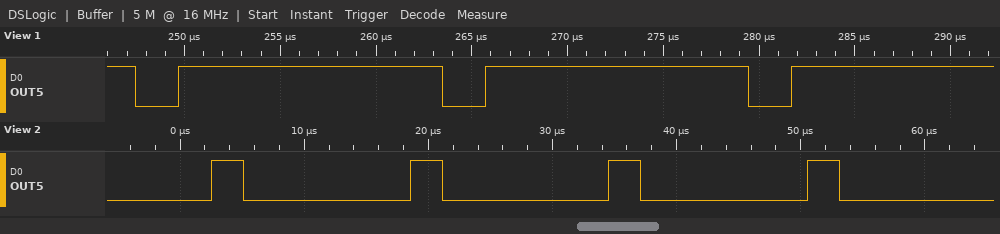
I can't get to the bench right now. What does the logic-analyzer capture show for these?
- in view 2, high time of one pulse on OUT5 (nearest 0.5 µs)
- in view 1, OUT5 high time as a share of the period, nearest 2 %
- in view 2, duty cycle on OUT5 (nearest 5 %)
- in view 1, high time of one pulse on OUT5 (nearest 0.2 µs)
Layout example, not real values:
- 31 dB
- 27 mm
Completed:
- 2.5 µs
- 86 %
- 15 %
- 13.8 µs
